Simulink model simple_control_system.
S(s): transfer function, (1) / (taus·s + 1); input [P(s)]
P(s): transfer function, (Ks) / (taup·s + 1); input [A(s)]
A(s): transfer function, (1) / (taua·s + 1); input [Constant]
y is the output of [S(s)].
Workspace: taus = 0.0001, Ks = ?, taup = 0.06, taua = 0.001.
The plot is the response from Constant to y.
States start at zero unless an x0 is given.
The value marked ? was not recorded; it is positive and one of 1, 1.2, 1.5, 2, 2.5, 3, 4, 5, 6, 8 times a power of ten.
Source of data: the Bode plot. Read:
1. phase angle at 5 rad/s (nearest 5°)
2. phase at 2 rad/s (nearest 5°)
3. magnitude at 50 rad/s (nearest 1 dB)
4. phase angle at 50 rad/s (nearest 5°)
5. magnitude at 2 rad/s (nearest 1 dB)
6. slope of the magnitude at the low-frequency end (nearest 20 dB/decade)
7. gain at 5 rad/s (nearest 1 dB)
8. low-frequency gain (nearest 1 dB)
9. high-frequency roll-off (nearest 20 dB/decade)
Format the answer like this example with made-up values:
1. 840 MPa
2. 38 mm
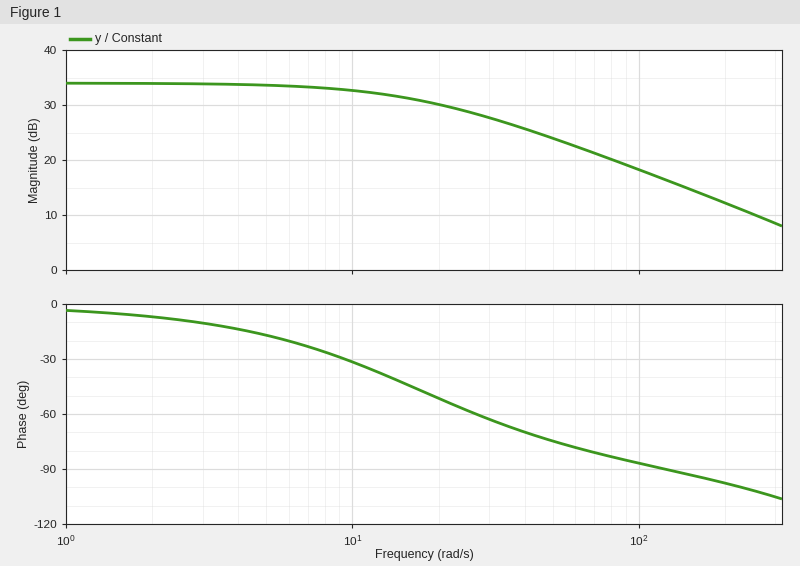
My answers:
1. -15°
2. -5°
3. 24 dB
4. -75°
5. 34 dB
6. 0 dB/decade
7. 34 dB
8. 34 dB
9. -20 dB/decade
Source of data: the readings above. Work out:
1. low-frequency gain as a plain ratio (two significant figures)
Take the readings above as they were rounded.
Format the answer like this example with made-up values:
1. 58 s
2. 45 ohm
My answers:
1. 50
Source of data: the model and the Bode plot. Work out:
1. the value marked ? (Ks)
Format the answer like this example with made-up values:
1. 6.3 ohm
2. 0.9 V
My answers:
1. 50
